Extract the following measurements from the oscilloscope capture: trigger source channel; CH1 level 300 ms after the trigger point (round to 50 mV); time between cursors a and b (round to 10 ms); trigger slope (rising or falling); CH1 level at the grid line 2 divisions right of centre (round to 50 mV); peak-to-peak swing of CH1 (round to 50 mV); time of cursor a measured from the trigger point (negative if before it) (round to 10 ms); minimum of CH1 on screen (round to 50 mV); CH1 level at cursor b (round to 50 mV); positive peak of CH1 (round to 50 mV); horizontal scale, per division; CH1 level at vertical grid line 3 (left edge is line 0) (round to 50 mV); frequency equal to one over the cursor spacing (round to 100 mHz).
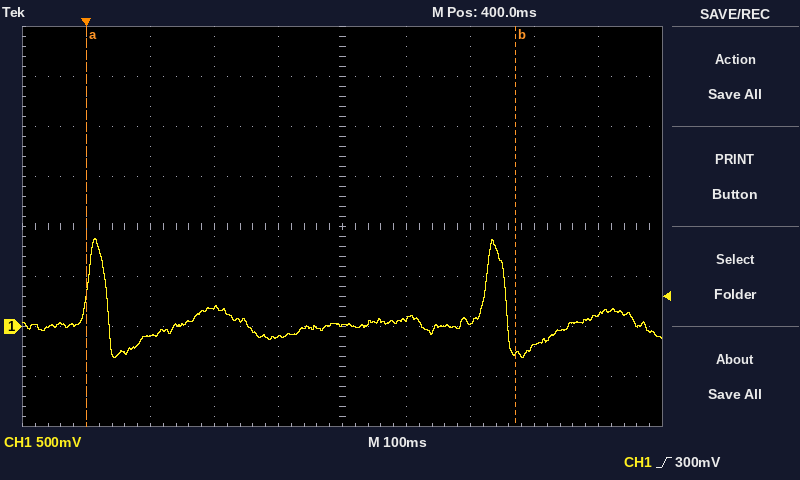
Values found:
CH1
-100 mV
670 ms
rising
50 mV
1.20 V
0 ms
-300 mV
-250 mV
900 mV
100 ms
200 mV
1.5 Hz
